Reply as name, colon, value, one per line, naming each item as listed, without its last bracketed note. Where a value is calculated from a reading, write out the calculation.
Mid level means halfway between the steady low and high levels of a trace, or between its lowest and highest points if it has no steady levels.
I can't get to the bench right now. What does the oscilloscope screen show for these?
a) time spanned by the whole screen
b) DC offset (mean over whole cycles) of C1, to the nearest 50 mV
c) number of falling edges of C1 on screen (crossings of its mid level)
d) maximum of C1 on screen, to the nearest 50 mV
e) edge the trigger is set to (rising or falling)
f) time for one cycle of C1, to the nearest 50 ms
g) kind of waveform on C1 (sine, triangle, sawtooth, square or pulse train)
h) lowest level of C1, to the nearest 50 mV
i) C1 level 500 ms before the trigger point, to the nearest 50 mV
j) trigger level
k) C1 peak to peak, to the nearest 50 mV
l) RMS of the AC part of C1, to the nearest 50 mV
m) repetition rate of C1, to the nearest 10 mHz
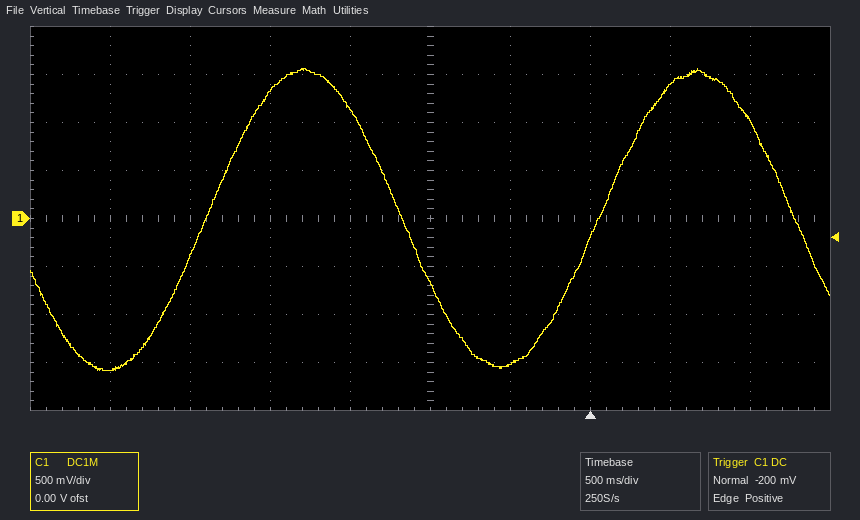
time spanned by the whole screen: 5 s
DC offset (mean over whole cycles) of C1, to the nearest 50 mV: (1.55 V + (-1.60 V)) / 2 ≈ 0 mV
number of falling edges of C1 on screen: 2
maximum of C1 on screen, to the nearest 50 mV: 1.55 V
edge the trigger is set to: rising
time for one cycle of C1, to the nearest 50 ms: 2.45 s
kind of waveform on C1: sine
lowest level of C1, to the nearest 50 mV: -1.60 V
C1 level 500 ms before the trigger point, to the nearest 50 mV: -1.50 V
trigger level: -200 mV
C1 peak to peak, to the nearest 50 mV: 1.55 V − (-1.60 V) = 3.15 V
RMS of the AC part of C1, to the nearest 50 mV: 3.15 V / (2√2) ≈ 1.11 V, so 1.10 V to the nearest 50 mV
repetition rate of C1, to the nearest 10 mHz: 1 / 2.45 s ≈ 408 mHz, so 410 mHz to the nearest 10 mHz
